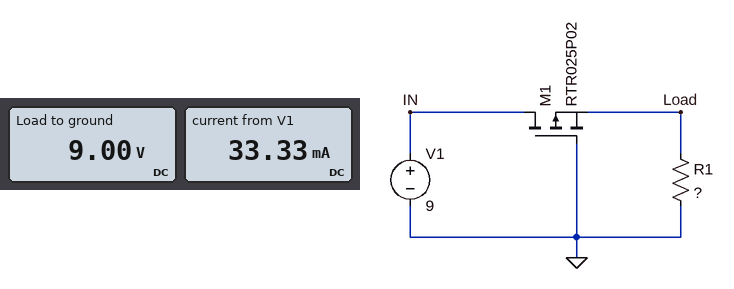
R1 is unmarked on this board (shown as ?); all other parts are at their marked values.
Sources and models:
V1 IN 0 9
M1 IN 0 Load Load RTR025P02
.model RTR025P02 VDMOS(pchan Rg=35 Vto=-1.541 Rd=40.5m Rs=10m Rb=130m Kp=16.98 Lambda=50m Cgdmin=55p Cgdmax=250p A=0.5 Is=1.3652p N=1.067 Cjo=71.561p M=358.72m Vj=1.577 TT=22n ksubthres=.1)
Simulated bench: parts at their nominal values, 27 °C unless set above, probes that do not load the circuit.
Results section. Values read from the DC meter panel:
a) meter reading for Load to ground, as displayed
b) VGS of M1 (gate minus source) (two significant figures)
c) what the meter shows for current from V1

9.00 V
-9.0 V
33.33 mA
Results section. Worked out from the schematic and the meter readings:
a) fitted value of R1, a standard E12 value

270 Ω
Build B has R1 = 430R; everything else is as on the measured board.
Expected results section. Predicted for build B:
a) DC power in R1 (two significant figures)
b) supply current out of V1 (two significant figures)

190 mW
21 mA
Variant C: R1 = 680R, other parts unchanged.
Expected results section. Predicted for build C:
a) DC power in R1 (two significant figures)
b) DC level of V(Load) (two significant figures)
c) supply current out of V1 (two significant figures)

120 mW
9.0 V
13 mA
